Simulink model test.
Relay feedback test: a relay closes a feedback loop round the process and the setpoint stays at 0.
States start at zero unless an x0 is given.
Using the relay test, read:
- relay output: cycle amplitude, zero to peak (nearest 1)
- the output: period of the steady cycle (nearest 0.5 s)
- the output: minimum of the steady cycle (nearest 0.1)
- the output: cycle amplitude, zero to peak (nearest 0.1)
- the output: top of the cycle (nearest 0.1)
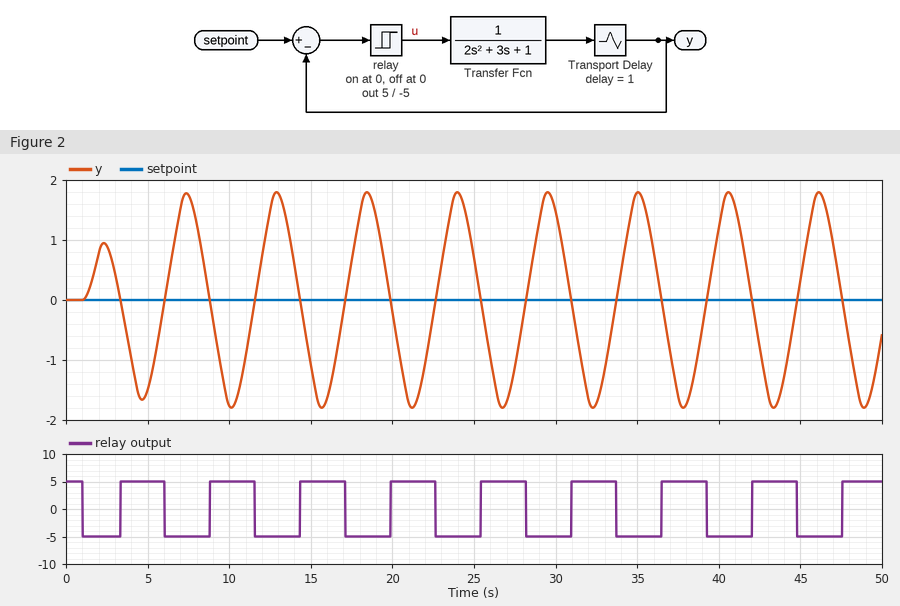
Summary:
5
5.5 s
-1.8
1.8
1.8
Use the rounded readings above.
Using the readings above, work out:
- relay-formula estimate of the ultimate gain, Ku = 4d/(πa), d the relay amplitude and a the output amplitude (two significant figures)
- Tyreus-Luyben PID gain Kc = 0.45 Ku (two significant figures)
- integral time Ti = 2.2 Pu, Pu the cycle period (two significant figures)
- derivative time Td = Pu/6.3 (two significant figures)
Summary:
3.5
1.6
12 s
0.87 s
